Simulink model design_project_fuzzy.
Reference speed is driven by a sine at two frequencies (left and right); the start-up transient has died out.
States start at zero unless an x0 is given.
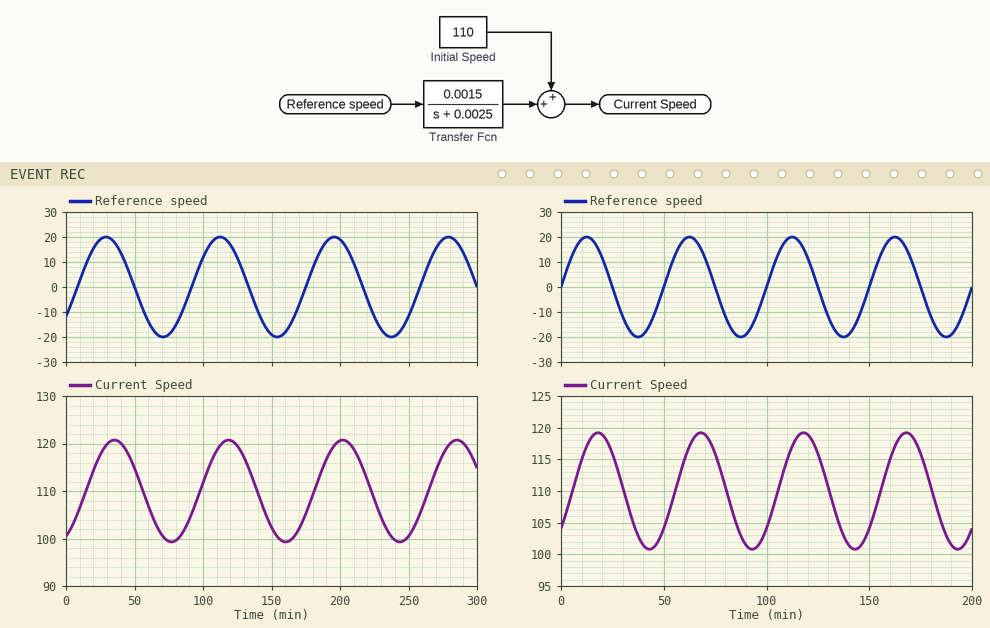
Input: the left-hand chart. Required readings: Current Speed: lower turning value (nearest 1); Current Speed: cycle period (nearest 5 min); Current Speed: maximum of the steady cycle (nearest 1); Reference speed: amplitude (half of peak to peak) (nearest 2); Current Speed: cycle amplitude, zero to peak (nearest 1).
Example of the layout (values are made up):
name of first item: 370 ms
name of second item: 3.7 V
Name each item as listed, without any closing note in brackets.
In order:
Current Speed: lower turning value: 99
Current Speed: cycle period: 85 min
Current Speed: maximum of the steady cycle: 121
Reference speed: amplitude (half of peak to peak): 20
Current Speed: cycle amplitude, zero to peak: 11
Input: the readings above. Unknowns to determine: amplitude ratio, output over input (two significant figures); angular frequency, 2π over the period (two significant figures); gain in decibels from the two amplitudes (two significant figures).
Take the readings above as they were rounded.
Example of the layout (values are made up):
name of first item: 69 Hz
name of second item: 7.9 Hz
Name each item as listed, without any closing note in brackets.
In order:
amplitude ratio, output over input: 0.55
angular frequency, 2π over the period: 0.074 rad/min
gain in decibels from the two amplitudes: -5.2 dB
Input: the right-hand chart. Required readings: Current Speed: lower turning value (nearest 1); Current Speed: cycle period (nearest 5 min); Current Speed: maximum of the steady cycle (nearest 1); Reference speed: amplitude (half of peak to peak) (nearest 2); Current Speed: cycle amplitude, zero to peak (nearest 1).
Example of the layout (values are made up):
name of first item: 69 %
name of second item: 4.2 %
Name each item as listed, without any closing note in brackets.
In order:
Current Speed: lower turning value: 101
Current Speed: cycle period: 50 min
Current Speed: maximum of the steady cycle: 119
Reference speed: amplitude (half of peak to peak): 20
Current Speed: cycle amplitude, zero to peak: 9
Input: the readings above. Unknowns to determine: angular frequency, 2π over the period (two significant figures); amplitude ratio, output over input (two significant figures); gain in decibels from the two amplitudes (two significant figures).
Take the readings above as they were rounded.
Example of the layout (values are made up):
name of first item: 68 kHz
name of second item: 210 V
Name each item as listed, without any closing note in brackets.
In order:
angular frequency, 2π over the period: 0.13 rad/min
amplitude ratio, output over input: 0.45
gain in decibels from the two amplitudes: -6.9 dB
